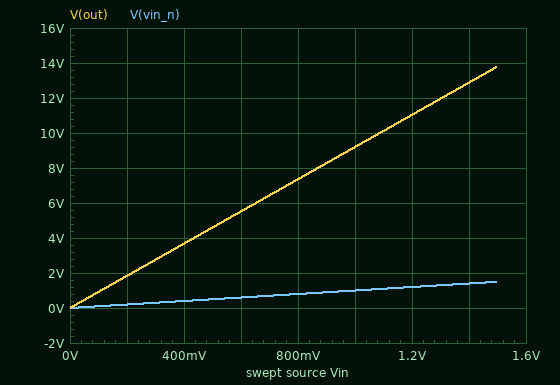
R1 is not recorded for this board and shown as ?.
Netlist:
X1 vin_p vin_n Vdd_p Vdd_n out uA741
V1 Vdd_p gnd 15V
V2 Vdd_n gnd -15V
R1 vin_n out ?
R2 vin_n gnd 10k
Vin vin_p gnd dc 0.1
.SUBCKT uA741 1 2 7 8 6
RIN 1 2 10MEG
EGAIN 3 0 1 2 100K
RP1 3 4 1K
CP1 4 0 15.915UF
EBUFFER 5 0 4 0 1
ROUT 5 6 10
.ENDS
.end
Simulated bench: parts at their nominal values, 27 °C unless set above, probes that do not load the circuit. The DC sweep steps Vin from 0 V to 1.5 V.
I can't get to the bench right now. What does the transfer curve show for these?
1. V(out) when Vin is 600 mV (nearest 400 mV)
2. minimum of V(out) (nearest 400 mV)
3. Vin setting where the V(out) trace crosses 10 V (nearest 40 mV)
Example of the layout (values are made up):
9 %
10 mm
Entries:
5.6 V
0 V
1.08 V
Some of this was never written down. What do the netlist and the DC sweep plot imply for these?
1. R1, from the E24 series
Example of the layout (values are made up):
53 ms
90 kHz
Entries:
82 kΩ
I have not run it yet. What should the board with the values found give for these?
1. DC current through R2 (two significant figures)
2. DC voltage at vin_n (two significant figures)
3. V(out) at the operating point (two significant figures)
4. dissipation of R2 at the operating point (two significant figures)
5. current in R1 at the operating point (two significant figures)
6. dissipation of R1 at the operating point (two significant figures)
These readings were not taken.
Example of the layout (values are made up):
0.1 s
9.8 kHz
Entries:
10 µA
100 mV
920 mV
1.0 µW
10 µA
8.2 µW
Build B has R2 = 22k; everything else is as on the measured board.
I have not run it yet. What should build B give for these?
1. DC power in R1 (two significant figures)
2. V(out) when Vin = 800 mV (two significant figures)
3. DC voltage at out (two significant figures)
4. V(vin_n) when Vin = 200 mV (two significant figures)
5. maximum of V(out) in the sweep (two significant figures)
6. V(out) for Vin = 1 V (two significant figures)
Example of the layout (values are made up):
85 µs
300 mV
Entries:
1.7 µW
3.8 V
470 mV
200 mV
7.1 V
4.7 V
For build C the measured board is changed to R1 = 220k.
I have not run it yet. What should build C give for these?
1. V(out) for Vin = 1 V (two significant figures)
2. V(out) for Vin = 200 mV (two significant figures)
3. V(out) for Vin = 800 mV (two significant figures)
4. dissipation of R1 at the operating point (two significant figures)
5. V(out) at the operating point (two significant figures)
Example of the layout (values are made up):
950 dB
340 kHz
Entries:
23 V
4.6 V
18 V
22 µW
2.3 V
